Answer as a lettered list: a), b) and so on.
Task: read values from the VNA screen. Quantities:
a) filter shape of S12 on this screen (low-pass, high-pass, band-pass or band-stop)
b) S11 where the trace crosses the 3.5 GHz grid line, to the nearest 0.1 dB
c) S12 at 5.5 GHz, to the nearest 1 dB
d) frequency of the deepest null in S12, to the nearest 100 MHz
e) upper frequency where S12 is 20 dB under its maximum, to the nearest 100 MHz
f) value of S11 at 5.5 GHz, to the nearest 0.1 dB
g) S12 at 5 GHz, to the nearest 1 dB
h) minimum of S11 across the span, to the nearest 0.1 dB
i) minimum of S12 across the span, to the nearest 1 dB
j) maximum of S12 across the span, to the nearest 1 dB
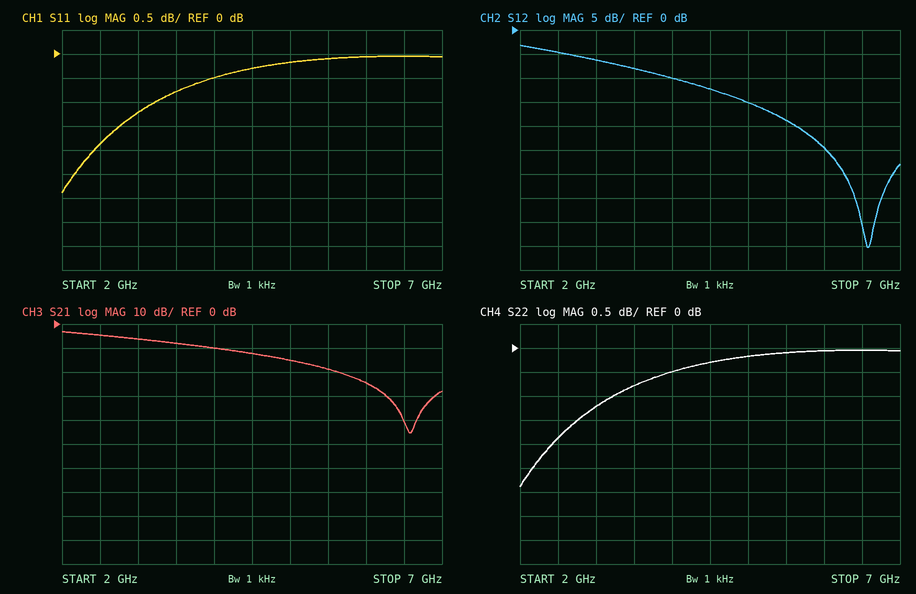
a) low-pass
b) -0.8 dB
c) -19 dB
d) 6.6 GHz
e) 5.9 GHz
f) -0.1 dB
g) -15 dB
h) -2.9 dB
i) -45 dB
j) -3 dB
